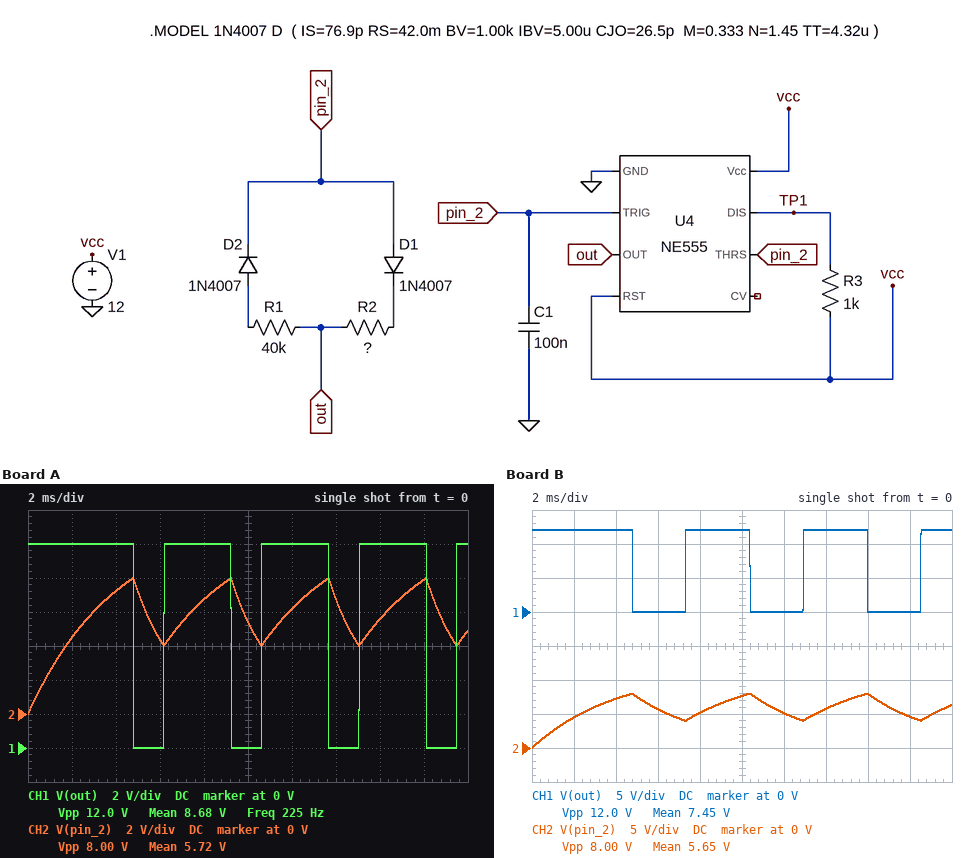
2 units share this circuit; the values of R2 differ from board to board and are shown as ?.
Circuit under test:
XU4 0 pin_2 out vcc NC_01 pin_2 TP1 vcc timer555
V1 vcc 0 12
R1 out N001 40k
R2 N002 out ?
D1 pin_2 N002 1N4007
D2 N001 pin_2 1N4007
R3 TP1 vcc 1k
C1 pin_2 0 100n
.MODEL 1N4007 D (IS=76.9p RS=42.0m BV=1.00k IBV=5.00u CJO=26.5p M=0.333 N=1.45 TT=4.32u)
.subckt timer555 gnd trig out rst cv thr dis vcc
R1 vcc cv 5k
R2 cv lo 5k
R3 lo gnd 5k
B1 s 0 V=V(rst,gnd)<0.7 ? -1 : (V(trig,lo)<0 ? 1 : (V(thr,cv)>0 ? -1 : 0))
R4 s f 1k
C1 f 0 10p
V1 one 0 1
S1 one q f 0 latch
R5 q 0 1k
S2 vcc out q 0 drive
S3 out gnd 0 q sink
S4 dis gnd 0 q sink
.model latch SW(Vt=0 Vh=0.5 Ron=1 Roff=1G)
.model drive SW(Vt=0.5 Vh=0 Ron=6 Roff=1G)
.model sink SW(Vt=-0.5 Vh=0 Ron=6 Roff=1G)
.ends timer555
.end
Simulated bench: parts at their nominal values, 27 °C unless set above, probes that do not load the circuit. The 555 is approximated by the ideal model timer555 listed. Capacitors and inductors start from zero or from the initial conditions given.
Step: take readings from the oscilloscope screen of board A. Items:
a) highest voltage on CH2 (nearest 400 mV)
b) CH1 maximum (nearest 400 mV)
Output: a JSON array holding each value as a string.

["8.0 V", "12.0 V"]
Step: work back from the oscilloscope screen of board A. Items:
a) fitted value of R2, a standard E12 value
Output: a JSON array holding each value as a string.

["18 kΩ"]
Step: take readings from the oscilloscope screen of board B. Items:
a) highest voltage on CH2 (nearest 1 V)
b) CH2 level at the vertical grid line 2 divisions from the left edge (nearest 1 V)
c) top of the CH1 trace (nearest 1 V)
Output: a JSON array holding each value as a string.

["8 V", "7 V", "12 V"]
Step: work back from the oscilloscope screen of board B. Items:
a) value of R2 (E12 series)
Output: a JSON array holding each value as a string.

["33 kΩ"]
